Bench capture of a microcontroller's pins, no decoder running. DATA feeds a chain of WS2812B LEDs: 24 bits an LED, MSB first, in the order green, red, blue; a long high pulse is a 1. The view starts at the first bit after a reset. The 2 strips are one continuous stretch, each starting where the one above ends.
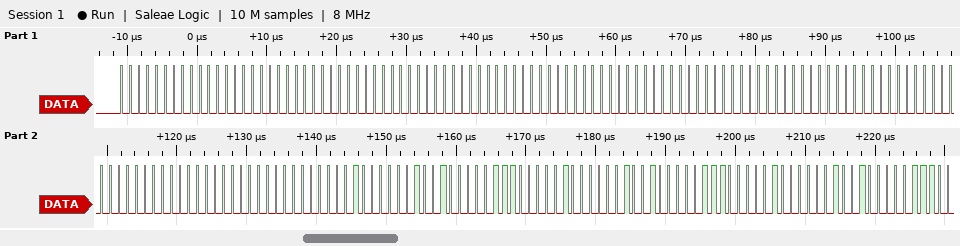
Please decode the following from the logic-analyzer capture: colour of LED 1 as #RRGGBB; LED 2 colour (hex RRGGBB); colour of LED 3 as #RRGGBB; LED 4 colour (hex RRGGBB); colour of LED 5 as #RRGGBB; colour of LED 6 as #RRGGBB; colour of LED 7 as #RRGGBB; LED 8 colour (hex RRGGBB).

#000000
#000000
#000000
#000000
#000000
#090407
#090407
#090407
